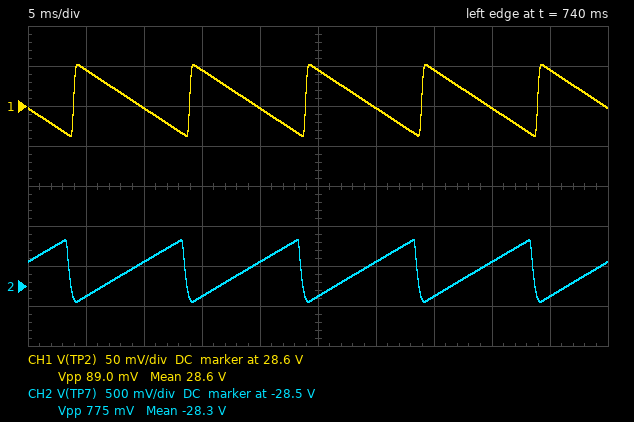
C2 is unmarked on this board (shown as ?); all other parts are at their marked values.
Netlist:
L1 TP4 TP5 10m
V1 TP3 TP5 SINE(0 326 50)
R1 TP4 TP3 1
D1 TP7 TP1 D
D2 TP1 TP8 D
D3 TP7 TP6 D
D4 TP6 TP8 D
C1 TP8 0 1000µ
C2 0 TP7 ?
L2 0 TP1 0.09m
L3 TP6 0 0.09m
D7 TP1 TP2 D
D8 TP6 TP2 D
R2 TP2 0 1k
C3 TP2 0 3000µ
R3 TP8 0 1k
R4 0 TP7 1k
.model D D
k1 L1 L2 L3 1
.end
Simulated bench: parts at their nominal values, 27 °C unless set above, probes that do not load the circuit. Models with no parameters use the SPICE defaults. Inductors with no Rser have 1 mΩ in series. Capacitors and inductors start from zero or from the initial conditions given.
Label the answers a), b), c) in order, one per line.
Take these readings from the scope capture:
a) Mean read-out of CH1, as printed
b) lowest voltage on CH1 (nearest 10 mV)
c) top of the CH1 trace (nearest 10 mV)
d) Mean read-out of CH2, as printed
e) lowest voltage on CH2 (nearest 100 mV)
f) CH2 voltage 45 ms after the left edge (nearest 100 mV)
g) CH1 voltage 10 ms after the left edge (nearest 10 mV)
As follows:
a) 28.6 V
b) 28.56 V
c) 28.65 V
d) -28.3 V
e) -28.7 V
f) -28.6 V
g) 28.60 V
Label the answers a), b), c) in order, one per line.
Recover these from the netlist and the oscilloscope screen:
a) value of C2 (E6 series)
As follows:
a) 330 µF
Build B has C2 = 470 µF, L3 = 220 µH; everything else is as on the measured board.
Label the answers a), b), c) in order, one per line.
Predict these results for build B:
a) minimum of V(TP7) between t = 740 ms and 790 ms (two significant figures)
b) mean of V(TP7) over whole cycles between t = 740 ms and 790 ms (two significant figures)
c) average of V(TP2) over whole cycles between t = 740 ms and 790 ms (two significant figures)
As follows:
a) -45 V
b) -44 V
c) 45 V
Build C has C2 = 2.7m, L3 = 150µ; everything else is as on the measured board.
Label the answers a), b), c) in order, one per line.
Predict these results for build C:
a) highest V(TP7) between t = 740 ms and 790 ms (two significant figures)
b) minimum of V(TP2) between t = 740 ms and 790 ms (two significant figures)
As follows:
a) -37 V
b) 37 V
